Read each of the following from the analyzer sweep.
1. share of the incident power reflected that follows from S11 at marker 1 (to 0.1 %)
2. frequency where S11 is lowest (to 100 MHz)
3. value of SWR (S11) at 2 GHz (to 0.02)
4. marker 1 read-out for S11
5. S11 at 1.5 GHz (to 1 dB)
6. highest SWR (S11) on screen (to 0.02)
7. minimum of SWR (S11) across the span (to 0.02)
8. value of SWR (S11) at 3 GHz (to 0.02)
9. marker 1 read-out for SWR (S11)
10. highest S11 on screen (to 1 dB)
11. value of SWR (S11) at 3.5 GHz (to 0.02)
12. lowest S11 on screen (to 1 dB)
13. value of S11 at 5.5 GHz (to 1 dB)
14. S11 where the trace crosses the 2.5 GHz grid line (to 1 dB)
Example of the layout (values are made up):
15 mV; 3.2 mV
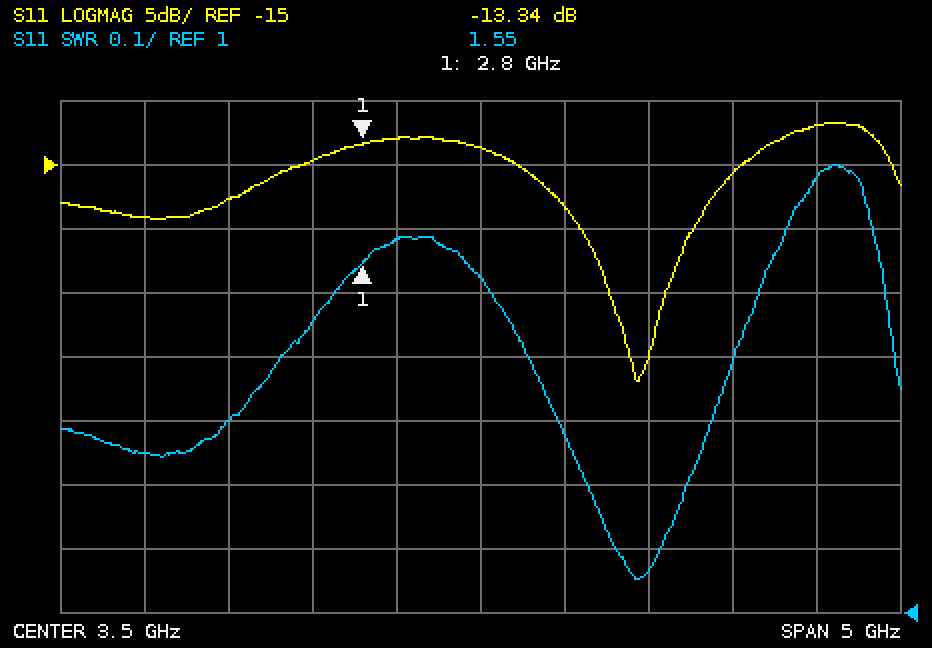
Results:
4.6 %; 4.4 GHz; 1.30; -13.34 dB; -19 dB; 1.70; 1.06; 1.58; 1.55; -12 dB; 1.52; -32 dB; -12 dB; -15 dB
